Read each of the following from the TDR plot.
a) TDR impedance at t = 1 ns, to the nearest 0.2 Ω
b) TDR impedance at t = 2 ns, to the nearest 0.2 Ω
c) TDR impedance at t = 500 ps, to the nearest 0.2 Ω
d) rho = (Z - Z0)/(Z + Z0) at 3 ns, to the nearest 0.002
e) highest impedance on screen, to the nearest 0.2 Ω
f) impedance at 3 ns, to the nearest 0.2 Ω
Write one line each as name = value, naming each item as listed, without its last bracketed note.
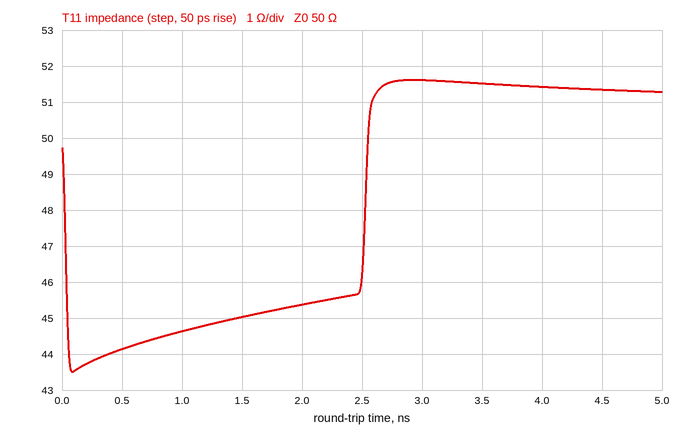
TDR impedance at t = 1 ns, to the nearest 0.2 Ω = 44.6 Ω
TDR impedance at t = 2 ns, to the nearest 0.2 Ω = 45.4 Ω
TDR impedance at t = 500 ps, to the nearest 0.2 Ω = 44.2 Ω
rho = (Z - Z0)/(Z + Z0) at 3 ns, to the nearest 0.002 = +0.016
highest impedance on screen, to the nearest 0.2 Ω = 51.6 Ω
impedance at 3 ns, to the nearest 0.2 Ω = 51.6 Ω
